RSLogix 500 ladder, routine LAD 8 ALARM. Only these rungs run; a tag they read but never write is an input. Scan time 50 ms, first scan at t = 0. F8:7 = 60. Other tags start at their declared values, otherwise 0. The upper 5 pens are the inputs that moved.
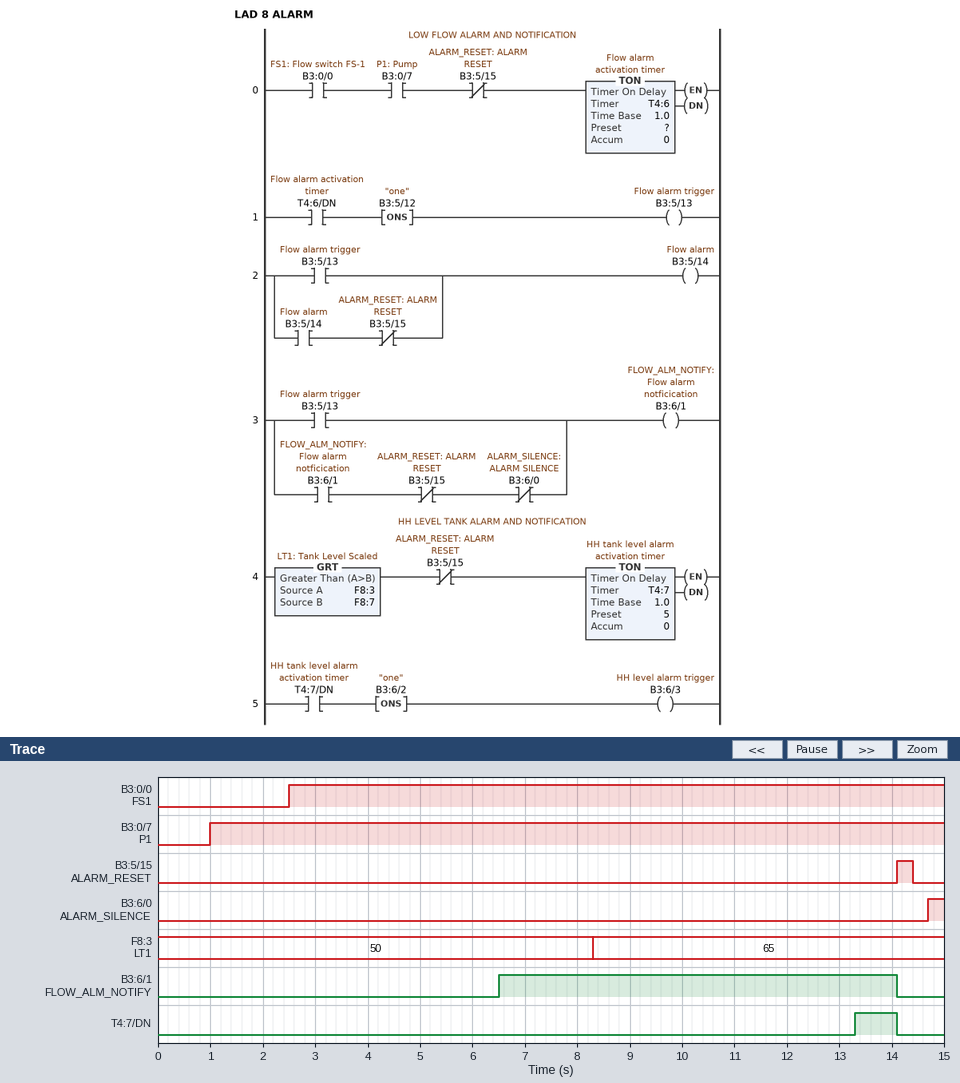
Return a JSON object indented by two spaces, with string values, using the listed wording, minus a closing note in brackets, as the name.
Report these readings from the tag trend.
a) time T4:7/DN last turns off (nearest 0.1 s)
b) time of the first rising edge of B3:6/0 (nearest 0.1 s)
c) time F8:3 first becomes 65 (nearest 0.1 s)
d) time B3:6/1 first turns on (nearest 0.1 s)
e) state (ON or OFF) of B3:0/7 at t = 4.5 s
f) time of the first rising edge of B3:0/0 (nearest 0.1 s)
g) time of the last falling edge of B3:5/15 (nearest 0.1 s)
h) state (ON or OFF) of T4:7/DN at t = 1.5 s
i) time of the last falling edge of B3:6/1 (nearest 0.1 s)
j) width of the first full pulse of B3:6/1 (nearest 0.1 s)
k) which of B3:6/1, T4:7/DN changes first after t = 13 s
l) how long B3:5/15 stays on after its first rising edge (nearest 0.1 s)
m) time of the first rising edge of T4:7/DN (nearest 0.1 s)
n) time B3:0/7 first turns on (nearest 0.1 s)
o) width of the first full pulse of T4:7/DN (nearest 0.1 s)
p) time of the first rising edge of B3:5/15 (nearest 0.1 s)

{
  "time T4:7/DN last turns off": "14.1 s",
  "time of the first rising edge of B3:6/0": "14.7 s",
  "time F8:3 first becomes 65": "8.3 s",
  "time B3:6/1 first turns on": "6.5 s",
  "state (ON or OFF) of B3:0/7 at t = 4.5 s": "ON",
  "time of the first rising edge of B3:0/0": "2.5 s",
  "time of the last falling edge of B3:5/15": "14.4 s",
  "state (ON or OFF) of T4:7/DN at t = 1.5 s": "OFF",
  "time of the last falling edge of B3:6/1": "14.1 s",
  "width of the first full pulse of B3:6/1": "7.6 s",
  "which of B3:6/1, T4:7/DN changes first after t = 13 s": "T4:7/DN",
  "how long B3:5/15 stays on after its first rising edge": "0.3 s",
  "time of the first rising edge of T4:7/DN": "13.3 s",
  "time B3:0/7 first turns on": "1.0 s",
  "width of the first full pulse of T4:7/DN": "0.8 s",
  "time of the first rising edge of B3:5/15": "14.1 s"
}
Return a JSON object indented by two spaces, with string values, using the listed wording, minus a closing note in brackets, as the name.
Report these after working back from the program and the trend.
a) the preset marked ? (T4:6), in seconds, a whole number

{
  "the preset marked ? (T4:6), in seconds, a whole number": "4 s"
}
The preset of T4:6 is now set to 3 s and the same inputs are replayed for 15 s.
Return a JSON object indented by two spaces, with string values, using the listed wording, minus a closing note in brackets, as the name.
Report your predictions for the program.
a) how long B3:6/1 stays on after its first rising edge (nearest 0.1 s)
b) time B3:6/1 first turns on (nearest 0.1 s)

{
  "how long B3:6/1 stays on after its first rising edge": "8.6 s",
  "time B3:6/1 first turns on": "5.5 s"
}
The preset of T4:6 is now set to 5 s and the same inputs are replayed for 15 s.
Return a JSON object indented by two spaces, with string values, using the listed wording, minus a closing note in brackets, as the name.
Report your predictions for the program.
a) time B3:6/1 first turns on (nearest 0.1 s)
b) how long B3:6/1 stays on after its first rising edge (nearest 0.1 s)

{
  "time B3:6/1 first turns on": "7.5 s",
  "how long B3:6/1 stays on after its first rising edge": "6.6 s"
}
